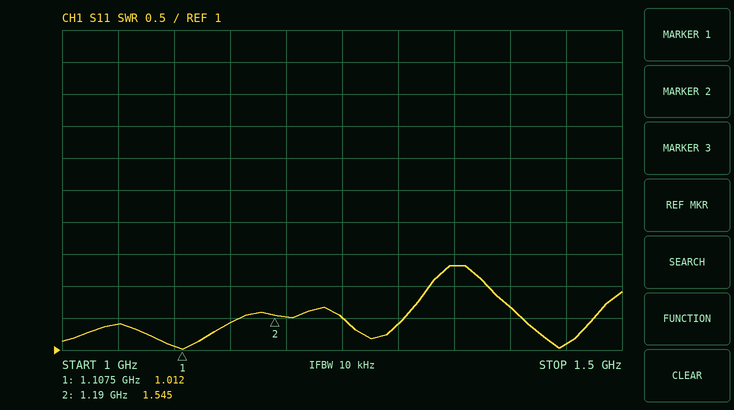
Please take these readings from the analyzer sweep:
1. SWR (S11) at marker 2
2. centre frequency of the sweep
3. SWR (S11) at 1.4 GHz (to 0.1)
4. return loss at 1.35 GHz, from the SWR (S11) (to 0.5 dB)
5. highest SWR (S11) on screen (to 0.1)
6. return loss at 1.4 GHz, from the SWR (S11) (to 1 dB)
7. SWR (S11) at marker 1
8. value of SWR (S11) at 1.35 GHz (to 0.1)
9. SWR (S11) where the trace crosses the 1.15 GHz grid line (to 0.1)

1.545
1.25 GHz
1.7
8.0 dB
2.3
12 dB
1.012
2.3
1.4
